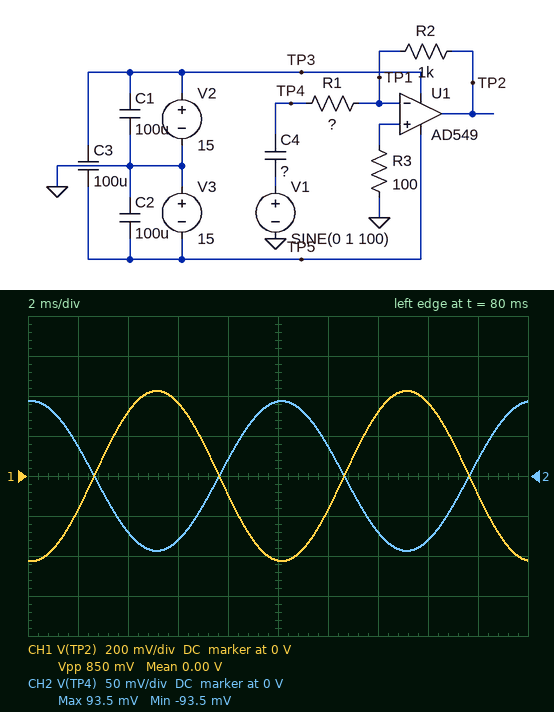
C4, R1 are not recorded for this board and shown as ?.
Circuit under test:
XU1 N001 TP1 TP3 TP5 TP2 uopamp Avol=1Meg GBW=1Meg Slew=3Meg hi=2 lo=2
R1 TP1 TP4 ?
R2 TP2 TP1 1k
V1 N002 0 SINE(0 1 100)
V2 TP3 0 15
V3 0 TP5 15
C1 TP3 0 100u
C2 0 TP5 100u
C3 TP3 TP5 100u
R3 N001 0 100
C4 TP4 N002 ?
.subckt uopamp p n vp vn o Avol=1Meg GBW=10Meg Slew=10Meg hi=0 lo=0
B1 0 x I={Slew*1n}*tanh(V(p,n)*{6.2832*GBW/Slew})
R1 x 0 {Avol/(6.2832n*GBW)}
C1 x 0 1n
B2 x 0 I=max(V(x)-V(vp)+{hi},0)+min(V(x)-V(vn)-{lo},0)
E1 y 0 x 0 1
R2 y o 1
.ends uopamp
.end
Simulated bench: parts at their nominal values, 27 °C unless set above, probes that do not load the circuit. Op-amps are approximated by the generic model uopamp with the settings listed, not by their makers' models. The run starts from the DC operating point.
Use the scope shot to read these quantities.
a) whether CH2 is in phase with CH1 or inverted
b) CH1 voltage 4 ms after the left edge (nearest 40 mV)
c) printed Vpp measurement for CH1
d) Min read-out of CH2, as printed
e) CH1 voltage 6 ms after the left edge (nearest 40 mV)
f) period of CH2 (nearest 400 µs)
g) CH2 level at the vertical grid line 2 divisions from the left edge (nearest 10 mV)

inverted
320 mV
850 mV
-93.5 mV
360 mV
10.0 ms
-70 mV
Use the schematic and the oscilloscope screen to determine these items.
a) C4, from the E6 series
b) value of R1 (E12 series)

680 nF
220 Ω
